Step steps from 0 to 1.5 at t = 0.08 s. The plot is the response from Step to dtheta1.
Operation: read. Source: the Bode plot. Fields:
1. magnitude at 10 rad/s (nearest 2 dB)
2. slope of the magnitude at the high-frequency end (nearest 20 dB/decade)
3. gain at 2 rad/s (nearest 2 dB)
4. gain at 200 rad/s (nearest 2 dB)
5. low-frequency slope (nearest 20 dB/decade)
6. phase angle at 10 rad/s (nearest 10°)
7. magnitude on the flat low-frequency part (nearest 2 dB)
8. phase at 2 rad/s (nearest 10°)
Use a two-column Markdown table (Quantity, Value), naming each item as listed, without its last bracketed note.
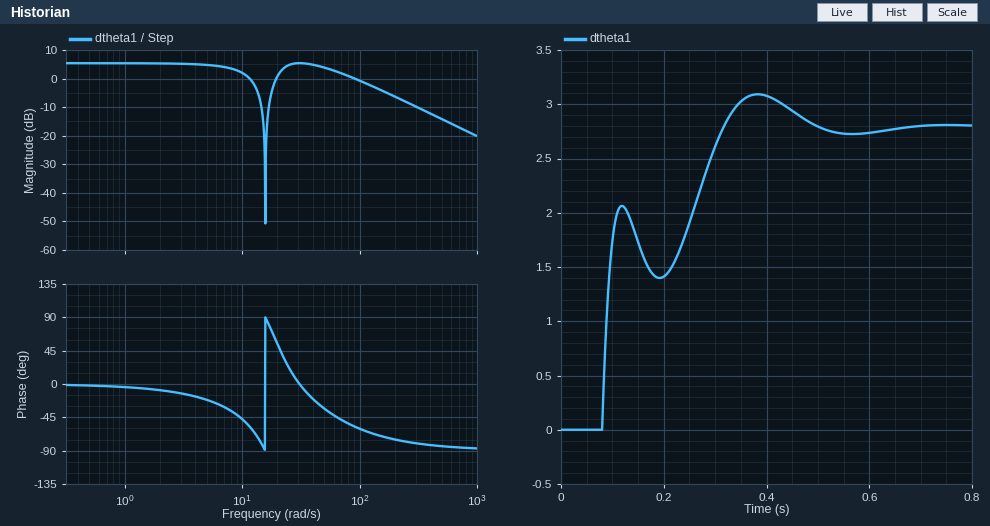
| Quantity | Value |
|---|---|
| magnitude at 10 rad/s | 2 dB |
| slope of the magnitude at the high-frequency end | -20 dB/decade |
| gain at 2 rad/s | 6 dB |
| gain at 200 rad/s | -6 dB |
| low-frequency slope | 0 dB/decade |
| phase angle at 10 rad/s | -50° |
| magnitude on the flat low-frequency part | 6 dB |
| phase at 2 rad/s | -10° |
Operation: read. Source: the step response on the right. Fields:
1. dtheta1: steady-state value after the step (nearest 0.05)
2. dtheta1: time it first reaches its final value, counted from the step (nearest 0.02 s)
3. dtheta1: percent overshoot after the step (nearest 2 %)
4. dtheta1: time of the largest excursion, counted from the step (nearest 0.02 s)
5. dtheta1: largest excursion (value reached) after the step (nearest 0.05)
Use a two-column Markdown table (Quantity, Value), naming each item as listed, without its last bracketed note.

| Quantity | Value |
|---|---|
| dtheta1: steady-state value after the step | 2.80 |
| dtheta1: time it first reaches its final value, counted from the step | 0.24 s |
| dtheta1: percent overshoot after the step | 10 % |
| dtheta1: time of the largest excursion, counted from the step | 0.30 s |
| dtheta1: largest excursion (value reached) after the step | 3.10 |
